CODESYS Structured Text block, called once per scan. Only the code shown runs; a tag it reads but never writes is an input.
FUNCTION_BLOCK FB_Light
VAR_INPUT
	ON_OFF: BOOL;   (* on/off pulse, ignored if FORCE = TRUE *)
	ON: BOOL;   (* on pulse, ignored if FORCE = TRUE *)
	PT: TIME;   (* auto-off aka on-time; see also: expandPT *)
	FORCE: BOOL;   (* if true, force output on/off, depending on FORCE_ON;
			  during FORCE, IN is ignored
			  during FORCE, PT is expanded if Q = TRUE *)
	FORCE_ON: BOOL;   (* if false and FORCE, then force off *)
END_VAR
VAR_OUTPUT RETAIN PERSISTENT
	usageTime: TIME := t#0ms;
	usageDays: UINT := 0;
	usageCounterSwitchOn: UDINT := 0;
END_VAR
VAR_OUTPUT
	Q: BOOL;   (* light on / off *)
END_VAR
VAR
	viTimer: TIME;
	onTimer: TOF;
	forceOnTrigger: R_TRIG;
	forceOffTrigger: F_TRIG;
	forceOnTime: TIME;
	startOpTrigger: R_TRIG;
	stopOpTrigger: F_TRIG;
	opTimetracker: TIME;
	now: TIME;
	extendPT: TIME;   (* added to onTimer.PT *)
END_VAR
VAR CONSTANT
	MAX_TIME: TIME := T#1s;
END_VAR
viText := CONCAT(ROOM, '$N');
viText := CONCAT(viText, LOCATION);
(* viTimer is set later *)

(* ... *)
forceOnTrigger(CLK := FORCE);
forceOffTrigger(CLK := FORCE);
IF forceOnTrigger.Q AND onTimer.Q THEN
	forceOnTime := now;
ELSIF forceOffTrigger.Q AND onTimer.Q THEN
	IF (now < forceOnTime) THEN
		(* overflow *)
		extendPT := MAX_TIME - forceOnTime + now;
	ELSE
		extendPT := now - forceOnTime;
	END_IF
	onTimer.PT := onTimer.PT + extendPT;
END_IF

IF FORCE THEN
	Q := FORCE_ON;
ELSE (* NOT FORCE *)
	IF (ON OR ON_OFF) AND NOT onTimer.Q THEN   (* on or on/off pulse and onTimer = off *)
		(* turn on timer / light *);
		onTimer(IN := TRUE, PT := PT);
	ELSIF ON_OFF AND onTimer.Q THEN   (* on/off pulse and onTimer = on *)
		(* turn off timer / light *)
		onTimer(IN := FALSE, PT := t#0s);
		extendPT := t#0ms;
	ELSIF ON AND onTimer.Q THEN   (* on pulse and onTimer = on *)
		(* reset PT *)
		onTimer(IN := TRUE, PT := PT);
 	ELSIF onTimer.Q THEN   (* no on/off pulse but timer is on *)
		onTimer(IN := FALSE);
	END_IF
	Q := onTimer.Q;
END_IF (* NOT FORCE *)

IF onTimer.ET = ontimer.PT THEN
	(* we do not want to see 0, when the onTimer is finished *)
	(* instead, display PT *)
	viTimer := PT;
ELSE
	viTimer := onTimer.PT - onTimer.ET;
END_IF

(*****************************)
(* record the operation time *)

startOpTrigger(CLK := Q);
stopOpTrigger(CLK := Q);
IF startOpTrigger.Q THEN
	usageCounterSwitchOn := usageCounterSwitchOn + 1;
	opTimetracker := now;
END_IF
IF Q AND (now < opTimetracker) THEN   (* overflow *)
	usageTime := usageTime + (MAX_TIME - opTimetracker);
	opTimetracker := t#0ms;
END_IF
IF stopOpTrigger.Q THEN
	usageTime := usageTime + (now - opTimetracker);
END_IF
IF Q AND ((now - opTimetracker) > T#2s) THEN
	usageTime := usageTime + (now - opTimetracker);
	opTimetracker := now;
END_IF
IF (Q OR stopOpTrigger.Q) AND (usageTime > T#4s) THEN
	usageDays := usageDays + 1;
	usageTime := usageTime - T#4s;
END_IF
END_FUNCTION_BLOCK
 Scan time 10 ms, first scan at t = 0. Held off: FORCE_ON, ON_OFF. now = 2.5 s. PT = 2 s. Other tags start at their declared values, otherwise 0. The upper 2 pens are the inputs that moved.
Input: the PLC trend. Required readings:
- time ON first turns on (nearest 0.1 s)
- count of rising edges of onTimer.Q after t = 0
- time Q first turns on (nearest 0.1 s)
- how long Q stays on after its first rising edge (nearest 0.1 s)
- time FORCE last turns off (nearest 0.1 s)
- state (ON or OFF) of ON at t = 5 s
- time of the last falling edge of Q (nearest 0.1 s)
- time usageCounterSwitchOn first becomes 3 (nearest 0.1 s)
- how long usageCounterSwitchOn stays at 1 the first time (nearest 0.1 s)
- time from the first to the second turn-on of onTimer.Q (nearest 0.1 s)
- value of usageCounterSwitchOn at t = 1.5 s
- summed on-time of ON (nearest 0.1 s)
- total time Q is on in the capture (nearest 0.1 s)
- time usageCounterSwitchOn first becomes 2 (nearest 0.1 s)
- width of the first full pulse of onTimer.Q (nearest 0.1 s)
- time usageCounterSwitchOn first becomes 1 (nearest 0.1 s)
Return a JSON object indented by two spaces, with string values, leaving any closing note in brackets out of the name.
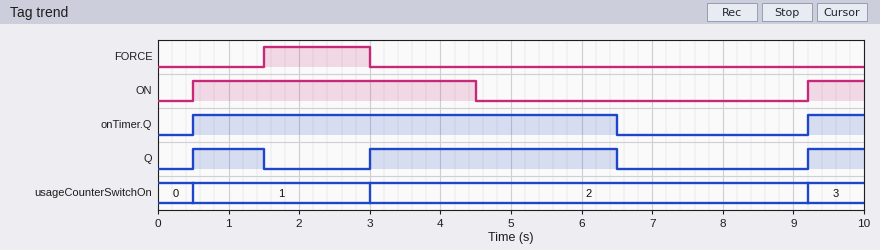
{
  "time ON first turns on": "0.5 s",
  "count of rising edges of onTimer.Q after t = 0": "2",
  "time Q first turns on": "0.5 s",
  "how long Q stays on after its first rising edge": "1.0 s",
  "time FORCE last turns off": "3.0 s",
  "state (ON or OFF) of ON at t = 5 s": "OFF",
  "time of the last falling edge of Q": "6.5 s",
  "time usageCounterSwitchOn first becomes 3": "9.2 s",
  "how long usageCounterSwitchOn stays at 1 the first time": "2.5 s",
  "time from the first to the second turn-on of onTimer.Q": "8.7 s",
  "value of usageCounterSwitchOn at t = 1.5 s": "1",
  "summed on-time of ON": "4.8 s",
  "total time Q is on in the capture": "5.3 s",
  "time usageCounterSwitchOn first becomes 2": "3.0 s",
  "width of the first full pulse of onTimer.Q": "6.0 s",
  "time usageCounterSwitchOn first becomes 1": "0.5 s"
}
